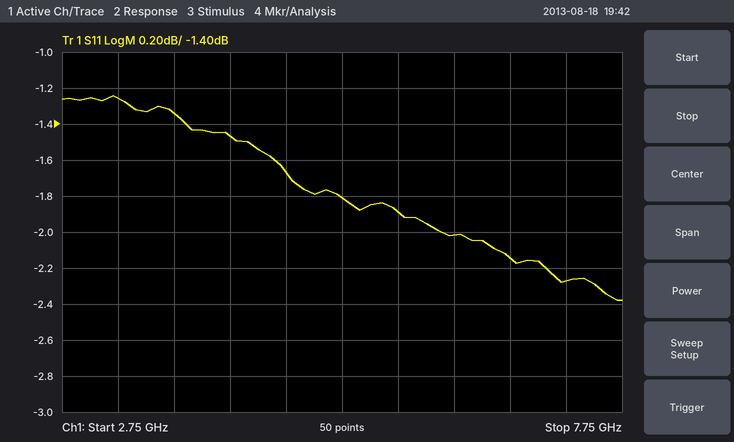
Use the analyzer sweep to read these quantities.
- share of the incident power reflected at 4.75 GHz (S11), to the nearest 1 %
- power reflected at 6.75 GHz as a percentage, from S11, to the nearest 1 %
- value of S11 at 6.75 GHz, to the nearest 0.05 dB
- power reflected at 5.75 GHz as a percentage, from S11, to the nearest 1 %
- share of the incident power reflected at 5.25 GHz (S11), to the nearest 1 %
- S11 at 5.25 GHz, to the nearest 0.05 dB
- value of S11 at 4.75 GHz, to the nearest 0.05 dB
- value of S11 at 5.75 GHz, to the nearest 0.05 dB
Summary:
68 %
61 %
-2.15 dB
65 %
66 %
-1.80 dB
-1.65 dB
-1.90 dB
